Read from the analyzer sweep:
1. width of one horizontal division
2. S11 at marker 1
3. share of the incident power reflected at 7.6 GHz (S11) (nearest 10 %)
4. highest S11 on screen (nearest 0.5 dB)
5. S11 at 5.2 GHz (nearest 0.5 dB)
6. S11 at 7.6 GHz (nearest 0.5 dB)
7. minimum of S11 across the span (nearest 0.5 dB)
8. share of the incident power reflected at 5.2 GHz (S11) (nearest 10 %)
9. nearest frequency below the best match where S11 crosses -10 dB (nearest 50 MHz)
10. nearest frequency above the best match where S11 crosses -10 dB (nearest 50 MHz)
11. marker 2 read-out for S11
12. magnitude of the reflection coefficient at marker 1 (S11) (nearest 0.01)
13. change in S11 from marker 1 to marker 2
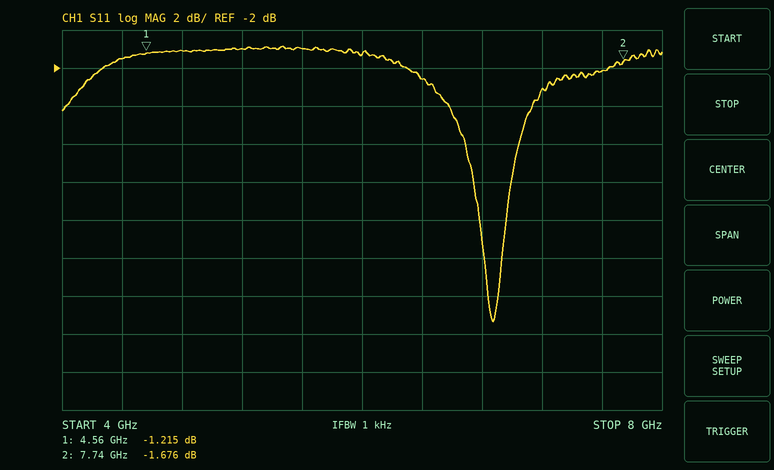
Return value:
400 MHz
-1.215 dB
60 %
-1.0 dB
-1.0 dB
-2.0 dB
-15.5 dB
80 %
6.80 GHz
6.95 GHz
-1.676 dB
0.87
-0.461 dB
